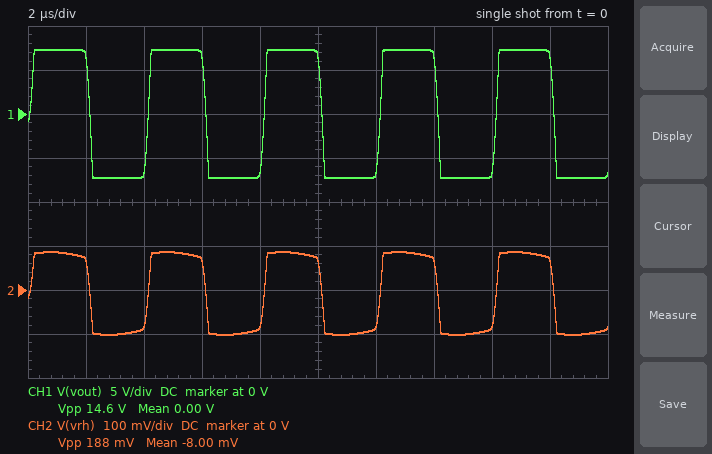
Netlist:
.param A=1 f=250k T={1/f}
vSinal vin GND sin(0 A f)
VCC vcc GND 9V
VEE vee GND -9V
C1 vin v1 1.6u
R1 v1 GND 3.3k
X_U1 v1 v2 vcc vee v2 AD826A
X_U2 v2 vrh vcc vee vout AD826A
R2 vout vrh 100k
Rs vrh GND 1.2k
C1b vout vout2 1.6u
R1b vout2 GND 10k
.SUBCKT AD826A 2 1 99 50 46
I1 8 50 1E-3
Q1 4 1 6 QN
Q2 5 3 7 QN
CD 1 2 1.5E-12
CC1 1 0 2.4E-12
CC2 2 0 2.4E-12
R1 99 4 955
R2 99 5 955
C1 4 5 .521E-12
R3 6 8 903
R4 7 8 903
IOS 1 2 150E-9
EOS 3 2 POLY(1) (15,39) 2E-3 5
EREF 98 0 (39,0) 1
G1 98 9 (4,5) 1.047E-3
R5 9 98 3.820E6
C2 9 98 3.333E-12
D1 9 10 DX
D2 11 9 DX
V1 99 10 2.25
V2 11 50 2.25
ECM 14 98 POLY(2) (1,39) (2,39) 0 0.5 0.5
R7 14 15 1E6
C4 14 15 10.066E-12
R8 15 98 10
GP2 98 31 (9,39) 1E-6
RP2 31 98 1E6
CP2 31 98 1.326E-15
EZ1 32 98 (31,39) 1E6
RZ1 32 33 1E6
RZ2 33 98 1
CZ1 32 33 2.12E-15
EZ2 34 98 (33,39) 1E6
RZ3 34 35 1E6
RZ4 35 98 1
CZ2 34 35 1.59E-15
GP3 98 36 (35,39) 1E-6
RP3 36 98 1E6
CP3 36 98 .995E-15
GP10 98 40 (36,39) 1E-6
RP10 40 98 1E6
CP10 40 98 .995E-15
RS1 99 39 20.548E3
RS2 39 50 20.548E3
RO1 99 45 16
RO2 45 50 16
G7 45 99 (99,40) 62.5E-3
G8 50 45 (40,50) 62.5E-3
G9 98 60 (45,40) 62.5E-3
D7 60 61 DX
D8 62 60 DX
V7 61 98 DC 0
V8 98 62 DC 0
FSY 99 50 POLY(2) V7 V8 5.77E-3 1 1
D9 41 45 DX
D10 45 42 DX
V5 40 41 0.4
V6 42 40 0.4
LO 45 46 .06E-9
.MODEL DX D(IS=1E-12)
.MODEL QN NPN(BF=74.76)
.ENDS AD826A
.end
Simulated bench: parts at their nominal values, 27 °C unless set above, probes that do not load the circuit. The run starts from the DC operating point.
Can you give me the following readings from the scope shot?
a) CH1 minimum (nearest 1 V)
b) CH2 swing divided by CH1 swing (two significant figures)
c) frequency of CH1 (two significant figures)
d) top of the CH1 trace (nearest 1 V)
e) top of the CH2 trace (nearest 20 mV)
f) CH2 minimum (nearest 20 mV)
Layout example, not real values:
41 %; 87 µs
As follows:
-7 V; 0.013; 250 kHz; 7 V; 80 mV; -100 mV
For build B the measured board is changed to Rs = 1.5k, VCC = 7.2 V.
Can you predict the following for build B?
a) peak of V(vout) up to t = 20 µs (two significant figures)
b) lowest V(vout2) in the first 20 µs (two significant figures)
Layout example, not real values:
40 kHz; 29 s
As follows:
5.5 V; -6.8 V
